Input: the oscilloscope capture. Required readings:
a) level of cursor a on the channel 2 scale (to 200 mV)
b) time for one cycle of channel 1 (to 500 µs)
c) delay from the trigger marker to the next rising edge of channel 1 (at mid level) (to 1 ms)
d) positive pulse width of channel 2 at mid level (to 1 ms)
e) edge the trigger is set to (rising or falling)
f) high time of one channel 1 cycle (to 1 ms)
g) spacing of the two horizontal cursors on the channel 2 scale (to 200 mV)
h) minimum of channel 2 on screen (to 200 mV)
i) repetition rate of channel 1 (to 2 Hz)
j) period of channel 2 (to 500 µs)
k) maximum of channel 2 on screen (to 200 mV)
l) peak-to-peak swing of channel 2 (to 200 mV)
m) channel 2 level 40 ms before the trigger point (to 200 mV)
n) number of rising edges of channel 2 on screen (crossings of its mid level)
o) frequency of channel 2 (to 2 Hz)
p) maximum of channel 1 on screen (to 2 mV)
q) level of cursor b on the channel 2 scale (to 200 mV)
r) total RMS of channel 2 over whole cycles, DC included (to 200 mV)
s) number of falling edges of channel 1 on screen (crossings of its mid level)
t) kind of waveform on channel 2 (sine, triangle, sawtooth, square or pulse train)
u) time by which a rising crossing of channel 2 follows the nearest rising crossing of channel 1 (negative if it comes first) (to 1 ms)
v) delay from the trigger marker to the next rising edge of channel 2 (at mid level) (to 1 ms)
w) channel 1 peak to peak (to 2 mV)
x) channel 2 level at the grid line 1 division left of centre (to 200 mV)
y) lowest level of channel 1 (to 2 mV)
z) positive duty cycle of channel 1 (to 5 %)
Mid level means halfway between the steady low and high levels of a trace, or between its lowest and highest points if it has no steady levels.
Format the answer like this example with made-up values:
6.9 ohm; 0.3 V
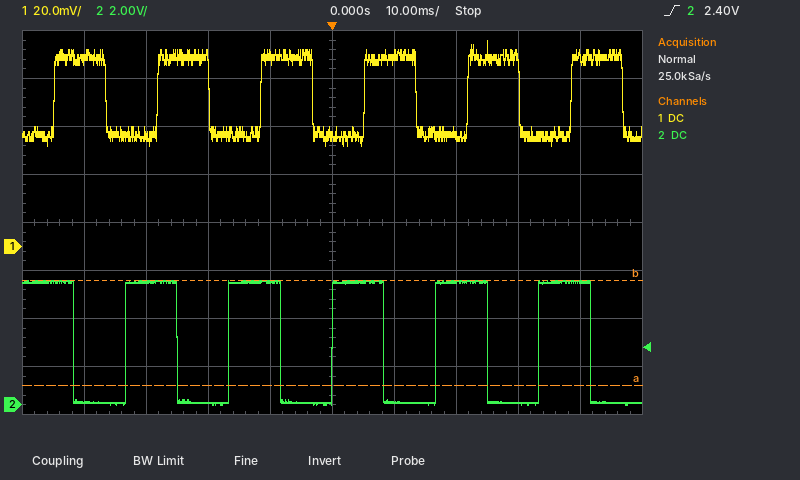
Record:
800 mV; 16.5 ms; 5 ms; 8 ms; rising; 8 ms; 4.4 V; 0.0 V; 60 Hz; 16.5 ms; 5.2 V; 5.2 V; 200 mV; 5; 60 Hz; 86 mV; 5.2 V; 3.6 V; 6; square; -5 ms; 17 ms; 44 mV; 5.2 V; 42 mV; 50 %
